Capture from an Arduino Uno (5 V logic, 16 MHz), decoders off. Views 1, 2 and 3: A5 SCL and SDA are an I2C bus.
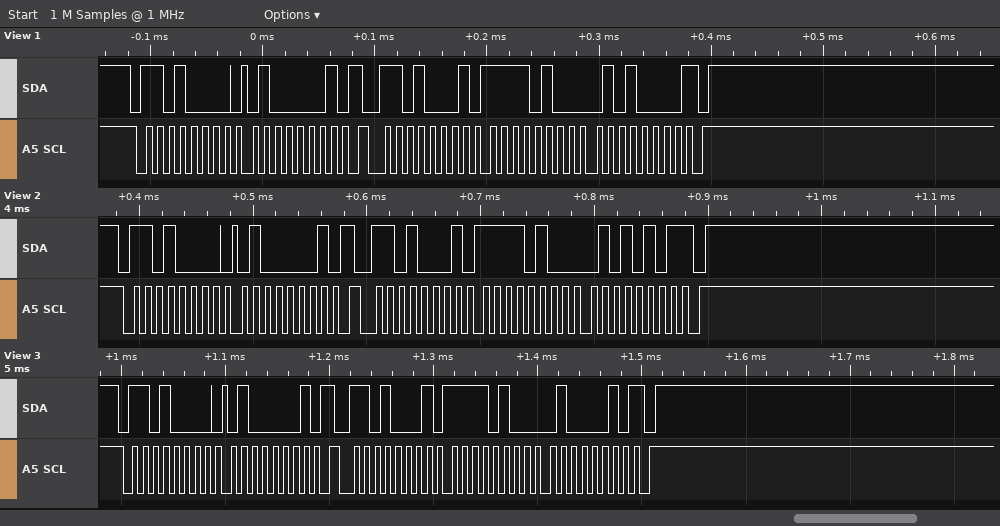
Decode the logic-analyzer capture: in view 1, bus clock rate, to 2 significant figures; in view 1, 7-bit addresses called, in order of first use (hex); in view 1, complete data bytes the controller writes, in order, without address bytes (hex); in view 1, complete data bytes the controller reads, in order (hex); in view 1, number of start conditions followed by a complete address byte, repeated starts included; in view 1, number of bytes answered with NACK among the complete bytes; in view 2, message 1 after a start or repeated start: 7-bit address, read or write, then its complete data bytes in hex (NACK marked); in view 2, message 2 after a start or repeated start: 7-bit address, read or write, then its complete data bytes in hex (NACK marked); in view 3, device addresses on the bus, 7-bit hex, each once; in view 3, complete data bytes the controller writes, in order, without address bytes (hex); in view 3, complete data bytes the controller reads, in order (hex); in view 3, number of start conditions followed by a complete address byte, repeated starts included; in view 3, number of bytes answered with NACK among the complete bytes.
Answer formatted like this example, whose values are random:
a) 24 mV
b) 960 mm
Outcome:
a) 100 kHz
b) 0x68
c) 41
d) F4 50
e) 2
f) 1
g) 0x68 write: 41
h) 0x68 read: F4 55 NACK
i) 0x68
j) 41
k) F4 42
l) 2
m) 1
